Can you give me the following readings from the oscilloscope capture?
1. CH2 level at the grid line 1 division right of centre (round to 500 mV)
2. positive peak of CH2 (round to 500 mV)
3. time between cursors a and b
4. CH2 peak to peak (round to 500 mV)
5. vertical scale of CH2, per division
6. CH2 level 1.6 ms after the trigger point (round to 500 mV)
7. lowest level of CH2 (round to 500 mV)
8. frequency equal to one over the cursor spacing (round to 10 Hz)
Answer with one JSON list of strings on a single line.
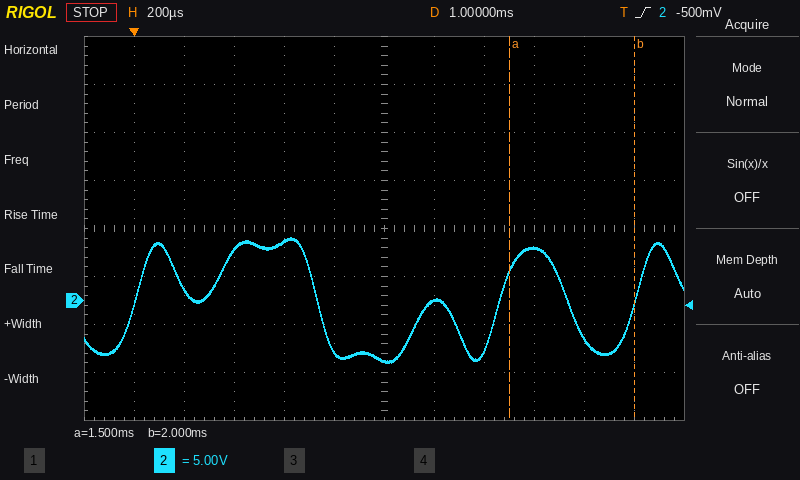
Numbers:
["0.0 V", "6.5 V", "500 µs", "13.0 V", "5 V", "5.5 V", "-6.5 V", "2.00 kHz"]
